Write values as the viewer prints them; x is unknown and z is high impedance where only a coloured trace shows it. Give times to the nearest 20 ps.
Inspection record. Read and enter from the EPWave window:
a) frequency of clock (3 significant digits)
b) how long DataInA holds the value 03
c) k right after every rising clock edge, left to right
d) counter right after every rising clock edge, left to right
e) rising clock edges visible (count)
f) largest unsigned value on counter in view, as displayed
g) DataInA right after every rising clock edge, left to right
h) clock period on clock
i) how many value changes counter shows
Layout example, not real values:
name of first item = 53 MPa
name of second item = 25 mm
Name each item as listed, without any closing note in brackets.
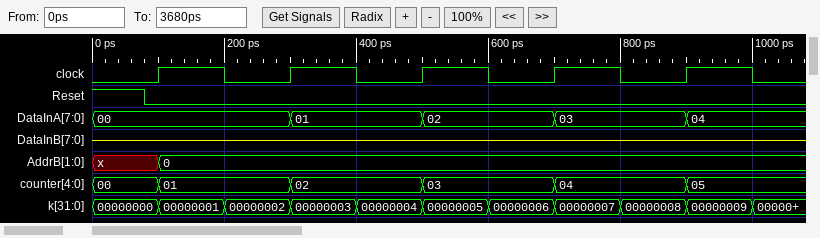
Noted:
frequency of clock = 5.00 GHz
how long DataInA holds the value 03 = 200 ps
k right after every rising clock edge, left to right = 00000001, 00000003, 00000005, 00000007, 00000009
counter right after every rising clock edge, left to right = 01, 02, 03, 04, 05
rising clock edges visible = 5
largest unsigned value on counter in view, as displayed = 05
DataInA right after every rising clock edge, left to right = 00, 01, 02, 03, 04
clock period on clock = 200 ps
how many value changes counter shows = 5
